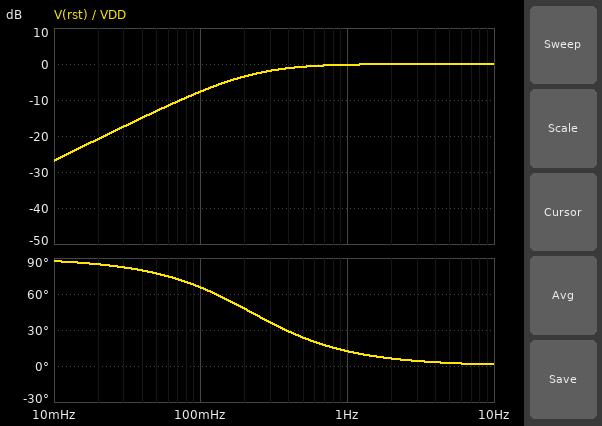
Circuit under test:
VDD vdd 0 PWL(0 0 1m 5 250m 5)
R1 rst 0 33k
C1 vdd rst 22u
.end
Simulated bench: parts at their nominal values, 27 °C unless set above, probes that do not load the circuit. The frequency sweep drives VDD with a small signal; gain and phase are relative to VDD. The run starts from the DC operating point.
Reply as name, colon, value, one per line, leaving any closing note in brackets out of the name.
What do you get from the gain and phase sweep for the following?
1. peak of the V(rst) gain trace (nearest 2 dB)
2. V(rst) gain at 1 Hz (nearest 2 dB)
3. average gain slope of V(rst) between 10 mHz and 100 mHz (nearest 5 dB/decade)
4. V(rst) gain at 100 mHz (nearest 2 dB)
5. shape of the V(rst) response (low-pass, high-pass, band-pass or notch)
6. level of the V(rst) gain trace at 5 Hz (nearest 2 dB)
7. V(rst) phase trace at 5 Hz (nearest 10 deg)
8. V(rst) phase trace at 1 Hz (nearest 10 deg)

peak of the V(rst) gain trace: 0 dB
V(rst) gain at 1 Hz: 0 dB
average gain slope of V(rst) between 10 mHz and 100 mHz: 20 dB/decade
V(rst) gain at 100 mHz: -8 dB
shape of the V(rst) response: high-pass
level of the V(rst) gain trace at 5 Hz: 0 dB
V(rst) phase trace at 5 Hz: 0 deg
V(rst) phase trace at 1 Hz: 10 deg
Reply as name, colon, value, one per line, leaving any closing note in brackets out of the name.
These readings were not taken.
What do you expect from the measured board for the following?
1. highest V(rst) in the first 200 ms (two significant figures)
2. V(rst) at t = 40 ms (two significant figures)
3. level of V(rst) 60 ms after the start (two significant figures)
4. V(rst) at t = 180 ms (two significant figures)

highest V(rst) in the first 200 ms: 5.0 V
V(rst) at t = 40 ms: 4.7 V
level of V(rst) 60 ms after the start: 4.6 V
V(rst) at t = 180 ms: 3.9 V
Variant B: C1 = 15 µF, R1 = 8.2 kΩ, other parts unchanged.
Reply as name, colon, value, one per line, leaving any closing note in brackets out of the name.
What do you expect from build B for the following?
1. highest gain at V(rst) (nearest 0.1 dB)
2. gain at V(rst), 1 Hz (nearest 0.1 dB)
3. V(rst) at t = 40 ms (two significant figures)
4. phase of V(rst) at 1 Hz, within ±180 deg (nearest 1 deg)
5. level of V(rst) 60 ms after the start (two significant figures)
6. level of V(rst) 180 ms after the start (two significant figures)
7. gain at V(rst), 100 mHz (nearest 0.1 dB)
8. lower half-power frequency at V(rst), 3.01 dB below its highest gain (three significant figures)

highest gain at V(rst): 0 dB
gain at V(rst), 1 Hz: -4.3 dB
V(rst) at t = 40 ms: 3.6 V
phase of V(rst) at 1 Hz, within ±180 deg: 52 deg
level of V(rst) 60 ms after the start: 3.1 V
level of V(rst) 180 ms after the start: 1.2 V
gain at V(rst), 100 mHz: -22.3 dB
lower half-power frequency at V(rst), 3.01 dB below its highest gain: 1.29 Hz
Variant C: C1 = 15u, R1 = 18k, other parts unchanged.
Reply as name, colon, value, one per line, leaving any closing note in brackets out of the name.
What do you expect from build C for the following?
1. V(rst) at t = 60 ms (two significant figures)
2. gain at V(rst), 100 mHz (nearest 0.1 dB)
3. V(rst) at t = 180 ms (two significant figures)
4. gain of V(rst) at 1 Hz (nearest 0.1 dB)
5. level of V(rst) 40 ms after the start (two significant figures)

V(rst) at t = 60 ms: 4.0 V
gain at V(rst), 100 mHz: -15.5 dB
V(rst) at t = 180 ms: 2.6 V
gain of V(rst) at 1 Hz: -1.3 dB
level of V(rst) 40 ms after the start: 4.3 V
